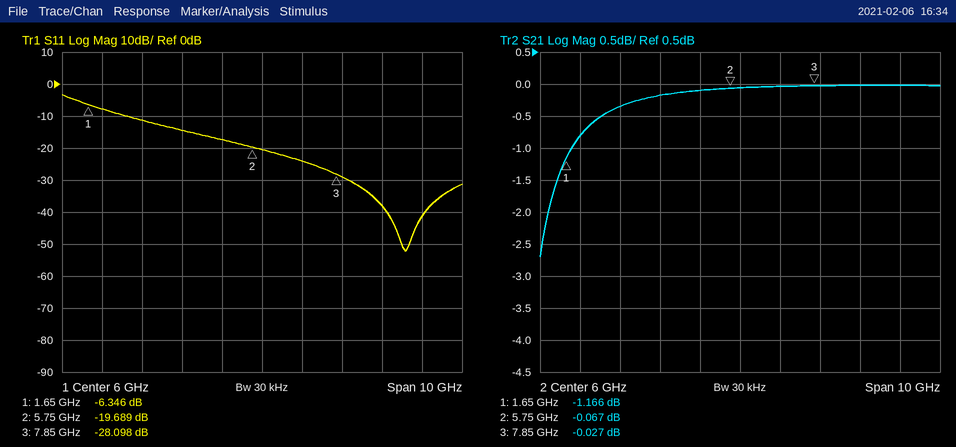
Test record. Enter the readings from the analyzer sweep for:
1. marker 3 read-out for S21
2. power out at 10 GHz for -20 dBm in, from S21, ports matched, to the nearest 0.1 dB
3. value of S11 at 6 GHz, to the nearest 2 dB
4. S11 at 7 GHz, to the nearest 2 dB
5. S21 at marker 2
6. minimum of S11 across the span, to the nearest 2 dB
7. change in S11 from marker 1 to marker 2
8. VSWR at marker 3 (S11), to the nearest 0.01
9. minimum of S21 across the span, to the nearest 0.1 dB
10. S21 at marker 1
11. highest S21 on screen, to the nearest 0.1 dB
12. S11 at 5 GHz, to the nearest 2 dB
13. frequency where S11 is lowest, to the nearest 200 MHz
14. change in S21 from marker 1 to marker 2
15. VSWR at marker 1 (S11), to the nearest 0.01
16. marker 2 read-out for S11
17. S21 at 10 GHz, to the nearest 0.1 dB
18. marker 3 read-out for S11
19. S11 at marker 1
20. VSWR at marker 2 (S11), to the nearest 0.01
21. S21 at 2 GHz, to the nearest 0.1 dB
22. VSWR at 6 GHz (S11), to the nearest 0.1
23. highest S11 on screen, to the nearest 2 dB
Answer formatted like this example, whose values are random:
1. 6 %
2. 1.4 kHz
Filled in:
1. -0.027 dB
2. -20.0 dBm
3. -20 dB
4. -24 dB
5. -0.067 dB
6. -52 dB
7. -13.343 dB
8. 1.08
9. -2.7 dB
10. -1.166 dB
11. 0.0 dB
12. -18 dB
13. 9.6 GHz
14. 1.099 dB
15. 2.86
16. -19.689 dB
17. 0.0 dB
18. -28.098 dB
19. -6.346 dB
20. 1.23
21. -0.8 dB
22. 1.2
23. -4 dB
